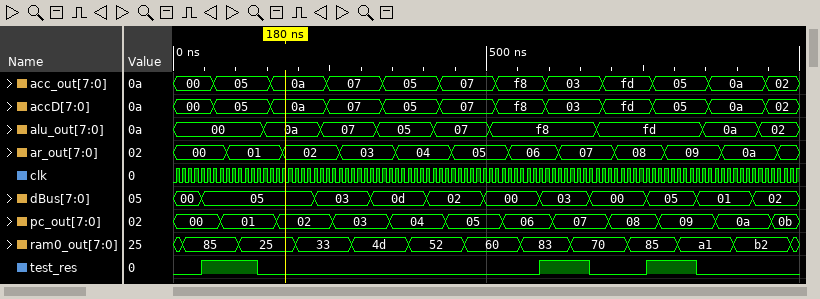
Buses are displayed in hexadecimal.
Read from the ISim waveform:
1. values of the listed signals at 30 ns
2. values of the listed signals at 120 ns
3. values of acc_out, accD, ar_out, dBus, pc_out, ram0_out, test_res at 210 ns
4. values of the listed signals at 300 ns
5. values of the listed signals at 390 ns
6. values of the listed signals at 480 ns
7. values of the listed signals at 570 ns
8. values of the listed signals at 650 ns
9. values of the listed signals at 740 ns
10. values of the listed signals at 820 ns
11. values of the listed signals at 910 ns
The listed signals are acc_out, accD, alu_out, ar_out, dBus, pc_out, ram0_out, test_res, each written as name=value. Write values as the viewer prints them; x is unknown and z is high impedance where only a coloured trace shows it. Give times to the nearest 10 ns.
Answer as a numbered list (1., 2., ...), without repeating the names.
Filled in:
1. acc_out=00, accD=00, alu_out=00, ar_out=00, dBus=00, pc_out=00, ram0_out=85, test_res=0
2. acc_out=05, accD=05, alu_out=00, ar_out=01, dBus=05, pc_out=01, ram0_out=25, test_res=1
3. acc_out=0a, accD=0a, ar_out=02, dBus=05, pc_out=02, ram0_out=33, test_res=0
4. acc_out=07, accD=07, alu_out=07, ar_out=03, dBus=03, pc_out=03, ram0_out=4d, test_res=0
5. acc_out=05, accD=05, alu_out=05, ar_out=04, dBus=0d, pc_out=04, ram0_out=52, test_res=0
6. acc_out=07, accD=07, alu_out=07, ar_out=05, dBus=02, pc_out=05, ram0_out=60, test_res=0
7. acc_out=f8, accD=f8, alu_out=f8, ar_out=06, dBus=00, pc_out=06, ram0_out=83, test_res=0
8. acc_out=03, accD=03, alu_out=f8, ar_out=07, dBus=03, pc_out=07, ram0_out=70, test_res=1
9. acc_out=fd, accD=fd, alu_out=fd, ar_out=08, dBus=00, pc_out=08, ram0_out=85, test_res=0
10. acc_out=05, accD=05, alu_out=fd, ar_out=09, dBus=05, pc_out=09, ram0_out=a1, test_res=1
11. acc_out=0a, accD=0a, alu_out=0a, ar_out=0a, dBus=01, pc_out=0a, ram0_out=b2, test_res=0
